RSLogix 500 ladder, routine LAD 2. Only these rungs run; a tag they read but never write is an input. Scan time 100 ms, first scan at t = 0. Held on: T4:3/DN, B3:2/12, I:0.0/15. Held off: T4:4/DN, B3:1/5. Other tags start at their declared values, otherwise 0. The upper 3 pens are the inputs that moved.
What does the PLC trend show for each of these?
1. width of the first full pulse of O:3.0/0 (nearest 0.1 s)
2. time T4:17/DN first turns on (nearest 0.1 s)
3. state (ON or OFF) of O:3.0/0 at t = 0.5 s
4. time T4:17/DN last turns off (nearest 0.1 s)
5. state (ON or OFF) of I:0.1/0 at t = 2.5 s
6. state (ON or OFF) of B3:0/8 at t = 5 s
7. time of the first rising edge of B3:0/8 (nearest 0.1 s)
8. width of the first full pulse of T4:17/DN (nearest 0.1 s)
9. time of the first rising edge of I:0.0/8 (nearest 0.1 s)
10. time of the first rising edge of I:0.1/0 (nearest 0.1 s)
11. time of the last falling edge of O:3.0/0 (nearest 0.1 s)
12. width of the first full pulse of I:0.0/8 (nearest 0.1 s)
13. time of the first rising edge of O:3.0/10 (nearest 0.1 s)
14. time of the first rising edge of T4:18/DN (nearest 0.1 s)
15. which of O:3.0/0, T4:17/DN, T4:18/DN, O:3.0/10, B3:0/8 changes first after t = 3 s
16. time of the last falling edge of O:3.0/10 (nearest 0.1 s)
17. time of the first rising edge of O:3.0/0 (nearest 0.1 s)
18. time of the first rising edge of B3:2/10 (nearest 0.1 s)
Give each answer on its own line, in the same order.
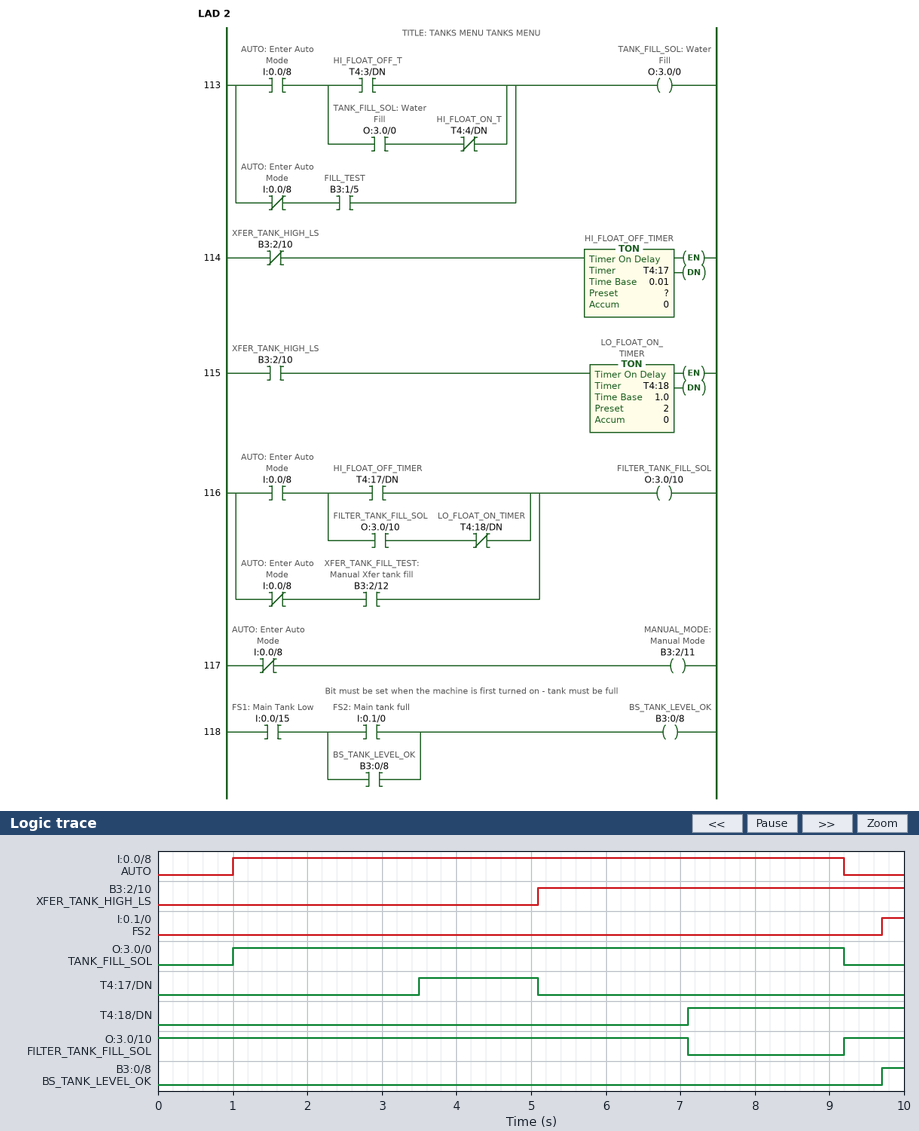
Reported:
8.2 s
3.5 s
OFF
5.1 s
OFF
OFF
9.7 s
1.6 s
1.0 s
9.7 s
9.2 s
8.2 s
9.2 s
7.1 s
T4:17/DN
7.1 s
1.0 s
5.1 s
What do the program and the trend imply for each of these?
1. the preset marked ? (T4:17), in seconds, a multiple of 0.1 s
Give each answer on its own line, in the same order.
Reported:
3.5 s
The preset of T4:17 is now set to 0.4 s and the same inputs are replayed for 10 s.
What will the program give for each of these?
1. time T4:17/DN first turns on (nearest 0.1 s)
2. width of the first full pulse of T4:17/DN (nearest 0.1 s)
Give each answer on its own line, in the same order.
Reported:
0.4 s
4.7 s
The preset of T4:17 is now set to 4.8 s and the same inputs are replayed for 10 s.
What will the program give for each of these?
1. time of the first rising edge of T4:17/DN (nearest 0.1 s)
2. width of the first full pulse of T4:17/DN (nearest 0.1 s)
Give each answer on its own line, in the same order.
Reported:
4.8 s
0.3 s
